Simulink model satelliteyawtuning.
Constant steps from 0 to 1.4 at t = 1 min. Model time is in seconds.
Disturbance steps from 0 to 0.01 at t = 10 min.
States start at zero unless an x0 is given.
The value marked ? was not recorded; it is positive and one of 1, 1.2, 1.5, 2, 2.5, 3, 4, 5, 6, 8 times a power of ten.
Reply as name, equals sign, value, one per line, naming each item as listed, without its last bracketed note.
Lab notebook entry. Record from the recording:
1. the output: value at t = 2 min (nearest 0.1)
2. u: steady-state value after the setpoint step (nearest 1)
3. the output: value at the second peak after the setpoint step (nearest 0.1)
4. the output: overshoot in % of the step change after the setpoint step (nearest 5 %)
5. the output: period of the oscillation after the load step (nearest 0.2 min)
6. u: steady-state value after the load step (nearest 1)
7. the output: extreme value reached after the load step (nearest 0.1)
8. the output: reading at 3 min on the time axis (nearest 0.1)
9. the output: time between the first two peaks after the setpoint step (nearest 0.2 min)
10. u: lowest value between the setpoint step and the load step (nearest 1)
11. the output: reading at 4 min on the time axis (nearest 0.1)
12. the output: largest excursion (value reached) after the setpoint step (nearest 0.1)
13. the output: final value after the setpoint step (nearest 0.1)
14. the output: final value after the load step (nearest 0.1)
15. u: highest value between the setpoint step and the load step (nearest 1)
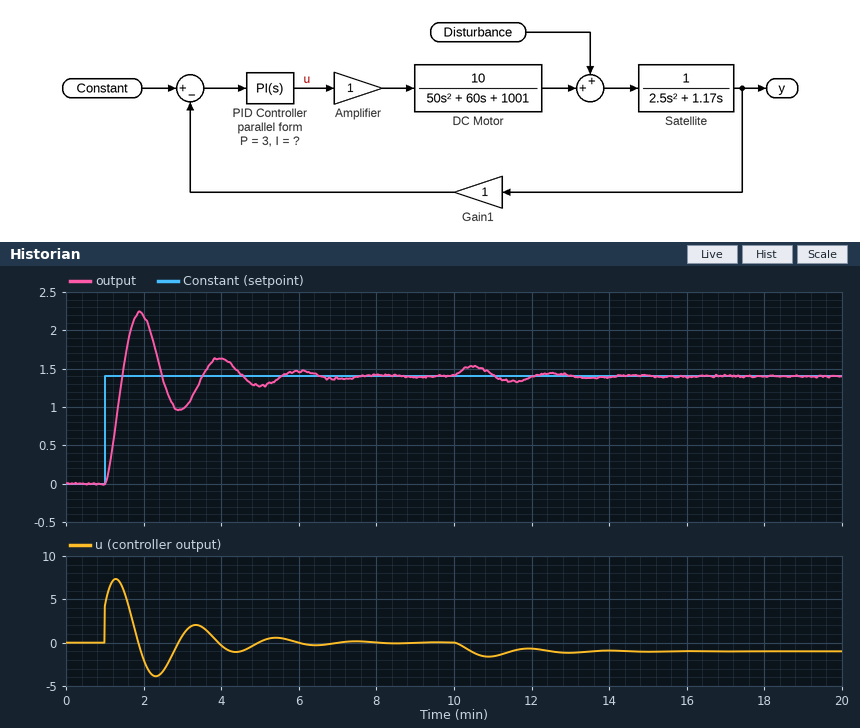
the output: value at t = 2 min = 2.2
u: steady-state value after the setpoint step = 0
the output: value at the second peak after the setpoint step = 1.6
the output: overshoot in % of the step change after the setpoint step = 60 %
the output: period of the oscillation after the load step = 2.0 min
u: steady-state value after the load step = -1
the output: extreme value reached after the load step = 1.5
the output: reading at 3 min on the time axis = 1.0
the output: time between the first two peaks after the setpoint step = 2.0 min
u: lowest value between the setpoint step and the load step = -4
the output: reading at 4 min on the time axis = 1.6
the output: largest excursion (value reached) after the setpoint step = 2.2
the output: final value after the setpoint step = 1.4
the output: final value after the load step = 1.4
u: highest value between the setpoint step and the load step = 7
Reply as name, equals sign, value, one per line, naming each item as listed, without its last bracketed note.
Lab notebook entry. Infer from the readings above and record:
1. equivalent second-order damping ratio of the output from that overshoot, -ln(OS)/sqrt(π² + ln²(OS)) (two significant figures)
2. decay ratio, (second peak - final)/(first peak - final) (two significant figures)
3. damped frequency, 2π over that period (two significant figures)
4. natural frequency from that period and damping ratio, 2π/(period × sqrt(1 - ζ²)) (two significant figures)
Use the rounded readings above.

equivalent second-order damping ratio of the output from that overshoot, -ln(OS)/sqrt(π² + ln²(OS)) = 0.16
decay ratio, (second peak - final)/(first peak - final) = 0.25
damped frequency, 2π over that period = 3.1 rad/min
natural frequency from that period and damping ratio, 2π/(period × sqrt(1 - ζ²)) = 3.2 rad/min
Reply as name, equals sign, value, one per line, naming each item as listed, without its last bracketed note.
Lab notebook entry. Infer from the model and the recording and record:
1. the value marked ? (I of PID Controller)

the value marked ? = 0.3
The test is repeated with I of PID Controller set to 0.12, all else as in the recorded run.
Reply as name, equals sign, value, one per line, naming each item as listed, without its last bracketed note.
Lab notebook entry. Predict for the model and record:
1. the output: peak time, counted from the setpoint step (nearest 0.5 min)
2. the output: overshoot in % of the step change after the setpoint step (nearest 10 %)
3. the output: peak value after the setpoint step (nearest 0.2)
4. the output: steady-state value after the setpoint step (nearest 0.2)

the output: peak time, counted from the setpoint step = 1.5 min
the output: overshoot in % of the step change after the setpoint step = 40 %
the output: peak value after the setpoint step = 2.0
the output: steady-state value after the setpoint step = 1.4
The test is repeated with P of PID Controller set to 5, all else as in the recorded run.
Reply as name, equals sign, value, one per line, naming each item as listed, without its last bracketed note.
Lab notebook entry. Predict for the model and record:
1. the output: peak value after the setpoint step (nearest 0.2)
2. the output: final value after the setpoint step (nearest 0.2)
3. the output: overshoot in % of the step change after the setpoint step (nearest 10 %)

the output: peak value after the setpoint step = 2.0
the output: final value after the setpoint step = 1.4
the output: overshoot in % of the step change after the setpoint step = 40 %
